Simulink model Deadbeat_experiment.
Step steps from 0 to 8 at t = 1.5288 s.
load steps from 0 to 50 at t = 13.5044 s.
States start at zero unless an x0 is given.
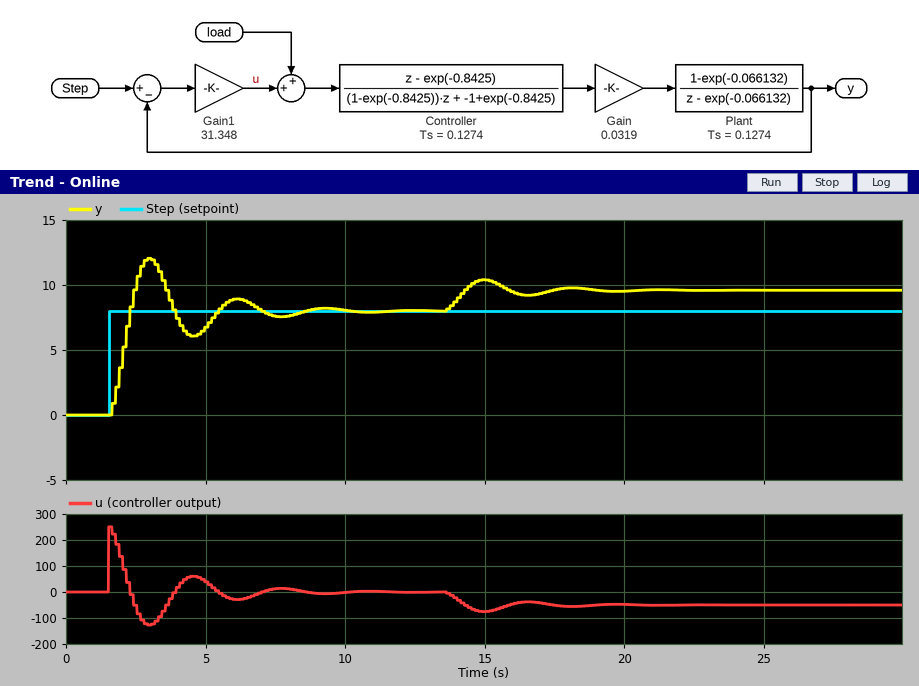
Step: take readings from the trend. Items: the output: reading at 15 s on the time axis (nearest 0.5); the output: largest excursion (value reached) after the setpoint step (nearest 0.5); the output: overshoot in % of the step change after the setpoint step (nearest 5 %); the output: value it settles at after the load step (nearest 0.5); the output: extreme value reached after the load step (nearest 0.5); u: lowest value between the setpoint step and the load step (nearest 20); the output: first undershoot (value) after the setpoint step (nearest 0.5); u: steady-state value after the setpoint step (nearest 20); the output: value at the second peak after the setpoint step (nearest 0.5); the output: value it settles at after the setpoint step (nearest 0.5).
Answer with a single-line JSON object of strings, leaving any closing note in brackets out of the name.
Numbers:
{"the output: reading at 15 s on the time axis": "10.5", "the output: largest excursion (value reached) after the setpoint step": "12.0", "the output: overshoot in % of the step change after the setpoint step": "50 %", "the output: value it settles at after the load step": "9.5", "the output: extreme value reached after the load step": "10.5", "u: lowest value between the setpoint step and the load step": "-120", "the output: first undershoot (value) after the setpoint step": "6.0", "u: steady-state value after the setpoint step": "0", "the output: value at the second peak after the setpoint step": "9.0", "the output: value it settles at after the setpoint step": "8.0"}
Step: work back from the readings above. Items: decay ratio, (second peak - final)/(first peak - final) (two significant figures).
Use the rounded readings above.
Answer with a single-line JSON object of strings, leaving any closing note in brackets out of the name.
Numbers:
{"decay ratio, (second peak - final)/(first peak - final)": "0.25"}
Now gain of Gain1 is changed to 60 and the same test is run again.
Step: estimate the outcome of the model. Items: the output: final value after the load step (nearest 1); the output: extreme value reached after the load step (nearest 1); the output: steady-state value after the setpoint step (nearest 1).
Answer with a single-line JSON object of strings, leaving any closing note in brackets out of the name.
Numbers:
{"the output: final value after the load step": "9", "the output: extreme value reached after the load step": "9", "the output: steady-state value after the setpoint step": "8"}
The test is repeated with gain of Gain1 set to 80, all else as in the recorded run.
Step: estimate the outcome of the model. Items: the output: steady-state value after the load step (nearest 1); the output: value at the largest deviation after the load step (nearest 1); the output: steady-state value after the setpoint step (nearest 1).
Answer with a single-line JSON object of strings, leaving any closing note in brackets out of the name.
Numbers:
{"the output: steady-state value after the load step": "9", "the output: value at the largest deviation after the load step": "9", "the output: steady-state value after the setpoint step": "8"}
